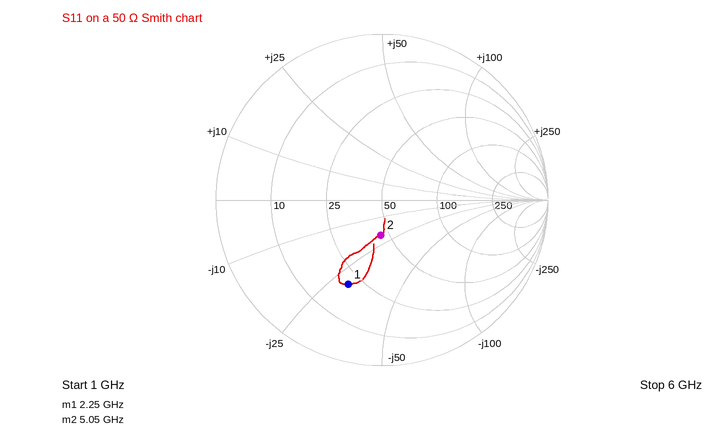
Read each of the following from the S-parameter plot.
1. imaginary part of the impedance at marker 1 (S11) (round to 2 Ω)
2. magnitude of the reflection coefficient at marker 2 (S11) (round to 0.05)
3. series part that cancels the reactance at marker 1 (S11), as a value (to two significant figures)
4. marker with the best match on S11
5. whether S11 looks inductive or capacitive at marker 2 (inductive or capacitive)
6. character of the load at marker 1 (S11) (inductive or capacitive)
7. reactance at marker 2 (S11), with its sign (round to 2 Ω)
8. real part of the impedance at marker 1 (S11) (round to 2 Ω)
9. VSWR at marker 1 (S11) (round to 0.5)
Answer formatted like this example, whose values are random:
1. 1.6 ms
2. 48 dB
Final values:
1. -30 Ω
2. 0.20
3. 2.1 nH
4. marker 2
5. capacitive
6. capacitive
7. -20 Ω
8. 20 Ω
9. 3.5
